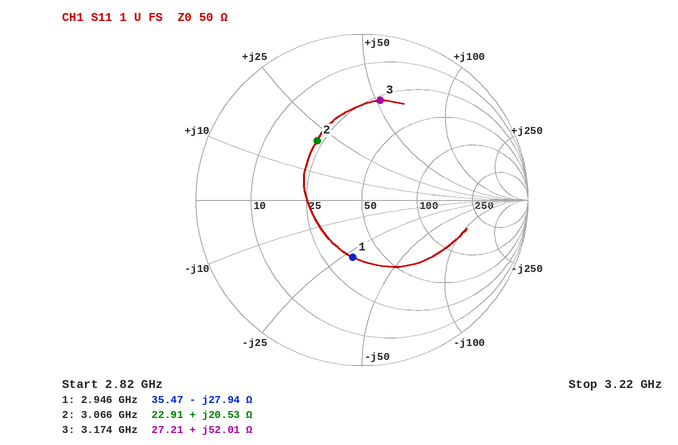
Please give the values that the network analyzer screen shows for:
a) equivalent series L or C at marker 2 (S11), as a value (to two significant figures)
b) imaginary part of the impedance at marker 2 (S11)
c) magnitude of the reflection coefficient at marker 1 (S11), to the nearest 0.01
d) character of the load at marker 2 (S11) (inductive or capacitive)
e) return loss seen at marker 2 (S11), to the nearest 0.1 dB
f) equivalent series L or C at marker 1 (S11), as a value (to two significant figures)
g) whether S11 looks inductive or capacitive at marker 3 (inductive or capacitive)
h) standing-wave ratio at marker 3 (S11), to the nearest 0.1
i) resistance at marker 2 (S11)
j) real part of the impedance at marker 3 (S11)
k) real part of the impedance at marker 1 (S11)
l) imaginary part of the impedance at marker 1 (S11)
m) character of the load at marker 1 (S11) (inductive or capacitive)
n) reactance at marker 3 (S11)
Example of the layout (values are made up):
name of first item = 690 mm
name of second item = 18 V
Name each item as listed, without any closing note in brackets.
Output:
equivalent series L or C at marker 2 (S11), as a value = 1.1 nH
imaginary part of the impedance at marker 2 = +20.53 Ω
magnitude of the reflection coefficient at marker 1 (S11), to the nearest 0.01 = 0.35
character of the load at marker 2 (S11) = inductive
return loss seen at marker 2 (S11), to the nearest 0.1 dB = 7.0 dB
equivalent series L or C at marker 1 (S11), as a value = 1.9 pF
whether S11 looks inductive or capacitive at marker 3 = inductive
standing-wave ratio at marker 3 (S11), to the nearest 0.1 = 4.1
resistance at marker 2 = 22.91 Ω
real part of the impedance at marker 3 = 27.21 Ω
real part of the impedance at marker 1 = 35.47 Ω
imaginary part of the impedance at marker 1 = -27.94 Ω
character of the load at marker 1 (S11) = capacitive
reactance at marker 3 = +52.01 Ω
